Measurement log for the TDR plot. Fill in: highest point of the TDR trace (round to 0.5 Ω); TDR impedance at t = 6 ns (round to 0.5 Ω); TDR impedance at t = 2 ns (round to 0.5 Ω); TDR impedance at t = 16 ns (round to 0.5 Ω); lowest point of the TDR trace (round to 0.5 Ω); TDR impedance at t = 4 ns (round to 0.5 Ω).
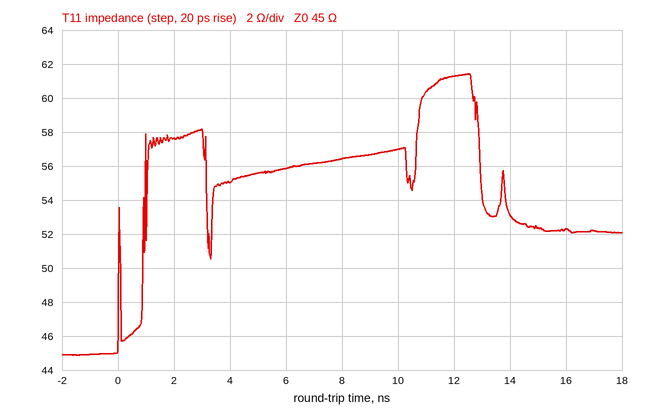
61.5 Ω
56.0 Ω
57.5 Ω
52.5 Ω
45.0 Ω
55.0 Ω
